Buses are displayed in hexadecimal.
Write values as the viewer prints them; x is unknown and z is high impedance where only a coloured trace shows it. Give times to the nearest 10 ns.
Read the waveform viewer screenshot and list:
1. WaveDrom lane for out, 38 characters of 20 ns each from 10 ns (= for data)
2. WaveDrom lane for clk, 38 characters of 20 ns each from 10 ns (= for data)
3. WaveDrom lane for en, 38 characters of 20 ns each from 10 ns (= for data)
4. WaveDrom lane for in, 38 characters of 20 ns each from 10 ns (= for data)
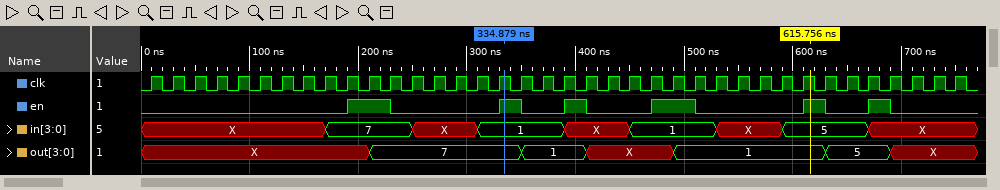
{name: 'out', wave: 'x.........=......=..x...=......=..x...', data: '7 1 1 5'}
{name: 'clk', wave: 'p.....................................'}
{name: 'en', wave: '0........1.0....10.10..1.0....10.10...'}
{name: 'in', wave: 'x.......=...x..=...x..=...x..=...x....', data: '7 1 1 5'}
